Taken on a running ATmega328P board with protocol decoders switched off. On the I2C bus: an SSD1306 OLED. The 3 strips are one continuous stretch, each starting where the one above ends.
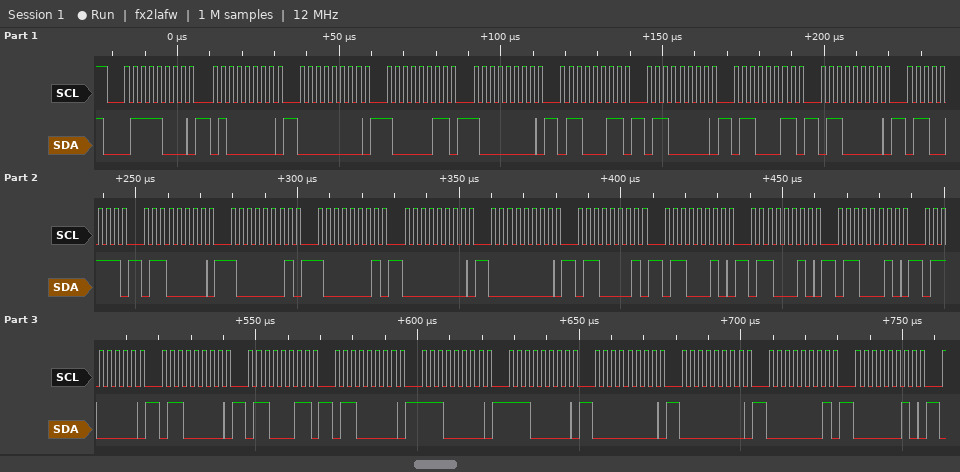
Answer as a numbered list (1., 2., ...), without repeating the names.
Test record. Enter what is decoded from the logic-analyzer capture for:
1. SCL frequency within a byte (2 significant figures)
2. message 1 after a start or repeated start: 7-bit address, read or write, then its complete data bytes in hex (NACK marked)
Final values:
1. 400 kHz
2. 0x3C write: 40 00 83 80 63 60 63 60 67 60 81 81 00 00 61 62 62 62 60 60 63 60 E0 E0 00 00 01 02
